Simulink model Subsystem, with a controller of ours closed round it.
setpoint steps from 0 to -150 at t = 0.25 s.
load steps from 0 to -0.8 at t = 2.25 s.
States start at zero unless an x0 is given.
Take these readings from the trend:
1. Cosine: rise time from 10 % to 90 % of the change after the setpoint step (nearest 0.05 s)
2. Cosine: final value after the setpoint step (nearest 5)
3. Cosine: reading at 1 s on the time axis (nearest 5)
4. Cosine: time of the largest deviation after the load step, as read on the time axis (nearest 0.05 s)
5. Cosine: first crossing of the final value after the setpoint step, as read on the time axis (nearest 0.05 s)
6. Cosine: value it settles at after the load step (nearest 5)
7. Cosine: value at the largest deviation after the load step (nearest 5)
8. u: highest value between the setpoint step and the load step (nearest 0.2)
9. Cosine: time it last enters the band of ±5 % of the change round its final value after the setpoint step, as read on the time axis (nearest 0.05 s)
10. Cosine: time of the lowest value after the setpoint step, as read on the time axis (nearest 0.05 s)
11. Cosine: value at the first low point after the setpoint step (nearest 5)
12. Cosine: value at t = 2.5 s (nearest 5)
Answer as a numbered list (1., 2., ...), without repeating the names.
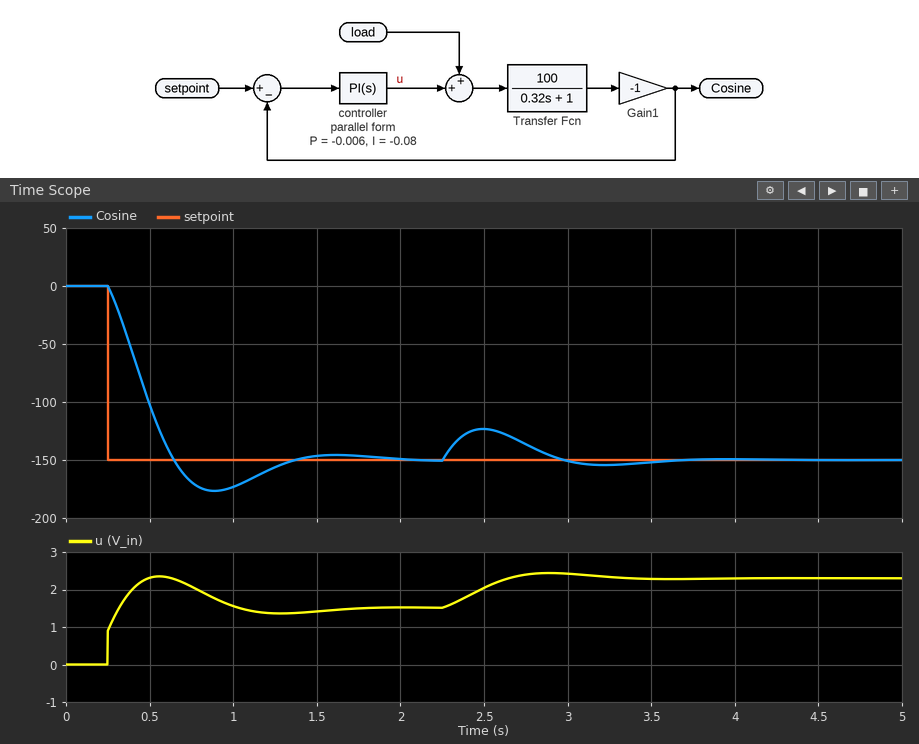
1. 0.30 s
2. -150
3. -175
4. 2.50 s
5. 0.65 s
6. -150
7. -125
8. 2.4
9. 1.25 s
10. 0.90 s
11. -175
12. -125
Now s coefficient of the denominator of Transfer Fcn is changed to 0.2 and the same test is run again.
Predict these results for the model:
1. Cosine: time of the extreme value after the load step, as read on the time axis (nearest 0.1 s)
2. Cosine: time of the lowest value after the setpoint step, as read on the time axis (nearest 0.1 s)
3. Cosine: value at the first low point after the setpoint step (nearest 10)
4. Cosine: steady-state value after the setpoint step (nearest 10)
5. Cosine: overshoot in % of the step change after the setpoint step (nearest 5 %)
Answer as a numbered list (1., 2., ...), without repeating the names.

1. 2.4 s
2. 0.8 s
3. -160
4. -150
5. 10 %
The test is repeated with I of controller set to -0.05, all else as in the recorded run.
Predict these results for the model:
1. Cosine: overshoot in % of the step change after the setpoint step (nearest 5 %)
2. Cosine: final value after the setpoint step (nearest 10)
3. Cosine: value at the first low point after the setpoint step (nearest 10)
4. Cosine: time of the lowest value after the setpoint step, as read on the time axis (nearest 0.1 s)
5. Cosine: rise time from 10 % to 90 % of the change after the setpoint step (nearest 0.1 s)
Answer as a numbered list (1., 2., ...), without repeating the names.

1. 10 %
2. -150
3. -160
4. 1.1 s
5. 0.4 s
